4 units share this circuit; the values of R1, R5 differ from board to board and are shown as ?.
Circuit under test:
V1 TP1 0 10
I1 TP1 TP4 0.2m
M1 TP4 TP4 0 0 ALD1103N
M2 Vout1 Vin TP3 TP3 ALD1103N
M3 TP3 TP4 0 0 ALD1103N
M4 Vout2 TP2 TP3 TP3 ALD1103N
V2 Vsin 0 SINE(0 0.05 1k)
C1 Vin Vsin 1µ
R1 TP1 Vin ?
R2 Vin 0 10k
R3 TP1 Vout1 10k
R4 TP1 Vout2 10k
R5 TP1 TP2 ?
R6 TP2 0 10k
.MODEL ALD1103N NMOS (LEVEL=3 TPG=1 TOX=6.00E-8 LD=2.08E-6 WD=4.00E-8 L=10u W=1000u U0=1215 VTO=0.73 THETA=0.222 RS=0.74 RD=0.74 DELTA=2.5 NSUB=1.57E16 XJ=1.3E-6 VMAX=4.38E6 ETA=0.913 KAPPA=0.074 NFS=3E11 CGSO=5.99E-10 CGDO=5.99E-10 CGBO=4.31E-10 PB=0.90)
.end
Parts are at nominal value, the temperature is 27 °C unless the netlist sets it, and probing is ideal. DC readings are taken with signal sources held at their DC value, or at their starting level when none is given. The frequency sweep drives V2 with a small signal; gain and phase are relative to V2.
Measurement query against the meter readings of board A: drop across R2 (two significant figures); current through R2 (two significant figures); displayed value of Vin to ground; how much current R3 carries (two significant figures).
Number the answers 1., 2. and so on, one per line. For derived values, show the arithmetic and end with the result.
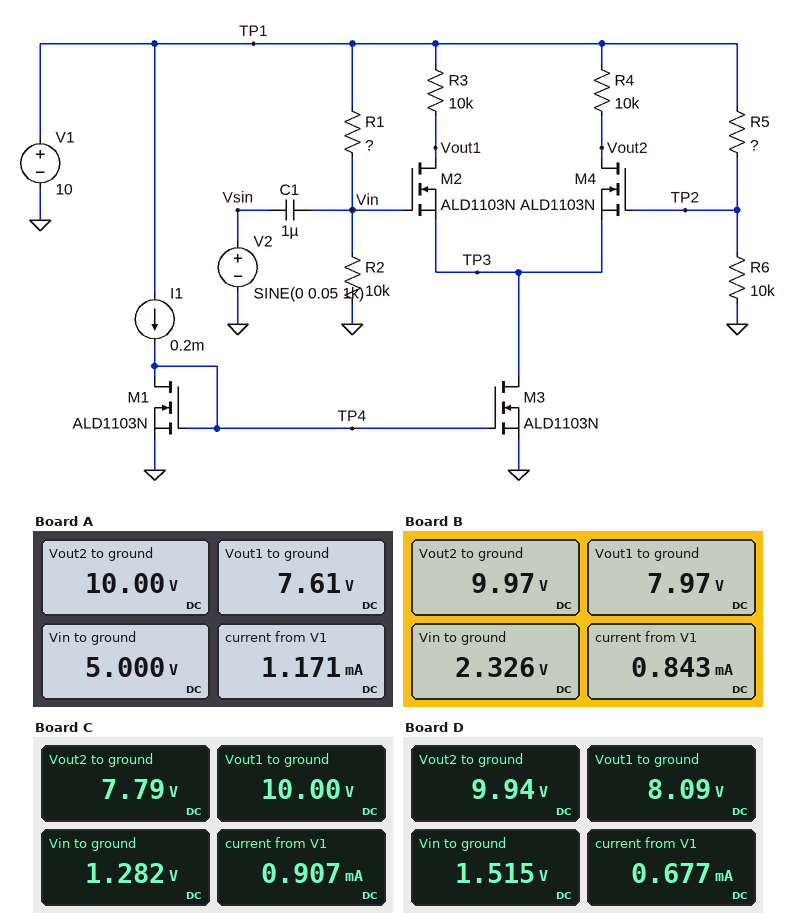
1. 5 V = 5.0 V
2. (5 V) / 10 kΩ = 500 µA
3. 5.000 V
4. (10 V - 7.61 V) / 10 kΩ = 240 µA
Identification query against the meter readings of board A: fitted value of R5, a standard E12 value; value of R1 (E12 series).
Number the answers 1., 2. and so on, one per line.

1. 33 kΩ
2. 10 kΩ
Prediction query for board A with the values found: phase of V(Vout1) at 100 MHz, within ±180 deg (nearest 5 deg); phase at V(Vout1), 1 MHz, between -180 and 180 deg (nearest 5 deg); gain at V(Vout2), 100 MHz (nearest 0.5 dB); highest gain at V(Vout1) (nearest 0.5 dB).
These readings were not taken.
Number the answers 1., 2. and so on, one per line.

1. 60 deg
2. -125 deg
3. -2.0 dB
4. 4.5 dB
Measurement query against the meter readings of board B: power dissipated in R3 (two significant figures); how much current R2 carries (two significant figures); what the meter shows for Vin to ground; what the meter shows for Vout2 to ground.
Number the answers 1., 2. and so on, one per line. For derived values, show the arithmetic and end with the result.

1. (10 V - 7.97 V)^2 / 10 kΩ = 410 µW
2. (2.326 V) / 10 kΩ = 230 µA
3. 2.326 V
4. 9.97 V
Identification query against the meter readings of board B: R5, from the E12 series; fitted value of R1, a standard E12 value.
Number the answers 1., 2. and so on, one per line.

1. 39 kΩ
2. 33 kΩ
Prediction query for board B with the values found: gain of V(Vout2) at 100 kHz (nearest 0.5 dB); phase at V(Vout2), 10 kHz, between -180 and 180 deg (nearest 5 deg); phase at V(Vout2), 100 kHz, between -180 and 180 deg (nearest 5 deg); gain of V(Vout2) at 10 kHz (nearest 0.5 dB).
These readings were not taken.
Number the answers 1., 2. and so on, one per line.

1. -6.5 dB
2. 0 deg
3. 0 deg
4. -6.5 dB
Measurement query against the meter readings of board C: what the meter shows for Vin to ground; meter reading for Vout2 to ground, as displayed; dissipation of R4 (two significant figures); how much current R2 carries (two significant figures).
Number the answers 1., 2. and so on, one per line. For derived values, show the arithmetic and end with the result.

1. 1.282 V
2. 7.79 V
3. (10 V - 7.79 V)^2 / 10 kΩ = 490 µW
4. (1.282 V) / 10 kΩ = 130 µA
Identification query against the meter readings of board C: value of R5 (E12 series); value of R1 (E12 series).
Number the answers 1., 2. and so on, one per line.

1. 18 kΩ
2. 68 kΩ
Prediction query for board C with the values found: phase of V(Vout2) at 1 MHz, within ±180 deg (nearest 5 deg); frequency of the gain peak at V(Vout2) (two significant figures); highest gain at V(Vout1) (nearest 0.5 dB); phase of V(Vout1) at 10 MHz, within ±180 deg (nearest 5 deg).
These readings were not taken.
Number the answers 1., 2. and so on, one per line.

1. 85 deg
2. 9.5 MHz
3. 0 dB
4. 70 deg
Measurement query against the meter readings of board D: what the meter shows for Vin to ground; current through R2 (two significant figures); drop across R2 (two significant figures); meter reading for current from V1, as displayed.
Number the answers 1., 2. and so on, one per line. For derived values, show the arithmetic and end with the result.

1. 1.515 V
2. (1.515 V) / 10 kΩ = 150 µA
3. 1.515 V = 1.5 V
4. 0.677 mA
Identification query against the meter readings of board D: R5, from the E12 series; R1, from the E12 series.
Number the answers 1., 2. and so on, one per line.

1. 68 kΩ
2. 56 kΩ
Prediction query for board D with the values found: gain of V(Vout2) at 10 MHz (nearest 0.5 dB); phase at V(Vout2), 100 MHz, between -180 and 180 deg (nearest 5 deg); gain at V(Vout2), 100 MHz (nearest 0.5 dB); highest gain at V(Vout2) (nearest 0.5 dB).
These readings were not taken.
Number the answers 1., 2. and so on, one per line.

1. -15.0 dB
2. 20 deg
3. -2.5 dB
4. -1.0 dB
